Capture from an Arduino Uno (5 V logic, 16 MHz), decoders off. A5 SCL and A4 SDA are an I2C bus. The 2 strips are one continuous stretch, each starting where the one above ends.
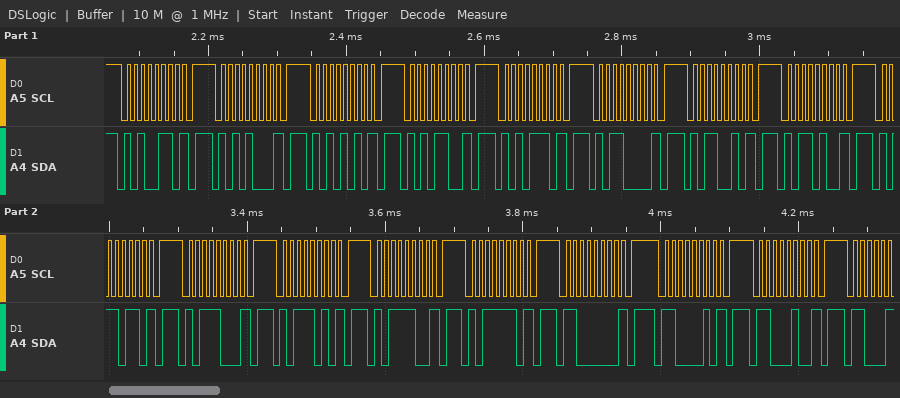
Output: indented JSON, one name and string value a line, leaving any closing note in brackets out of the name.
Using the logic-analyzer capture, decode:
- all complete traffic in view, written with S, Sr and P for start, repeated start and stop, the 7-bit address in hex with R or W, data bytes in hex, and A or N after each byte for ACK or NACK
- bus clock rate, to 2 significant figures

{
  "all complete traffic in view, written with S, Sr and P for start, repeated start and stop, the 7-bit address in hex with R or W, data bytes in hex, and A or N after each byte for ACK or NACK": "S 53W N P S 54W N P S 55W N P S 56W N P S 57W N P S 58W N P S 59W N P S 5AW N P S 5BW N P S 5CW N P S 5DW N P S 5EW N P S 5FW N P S 60W N P S 61W N P S 62W N P",
  "bus clock rate, to 2 significant figures": "100 kHz"
}
